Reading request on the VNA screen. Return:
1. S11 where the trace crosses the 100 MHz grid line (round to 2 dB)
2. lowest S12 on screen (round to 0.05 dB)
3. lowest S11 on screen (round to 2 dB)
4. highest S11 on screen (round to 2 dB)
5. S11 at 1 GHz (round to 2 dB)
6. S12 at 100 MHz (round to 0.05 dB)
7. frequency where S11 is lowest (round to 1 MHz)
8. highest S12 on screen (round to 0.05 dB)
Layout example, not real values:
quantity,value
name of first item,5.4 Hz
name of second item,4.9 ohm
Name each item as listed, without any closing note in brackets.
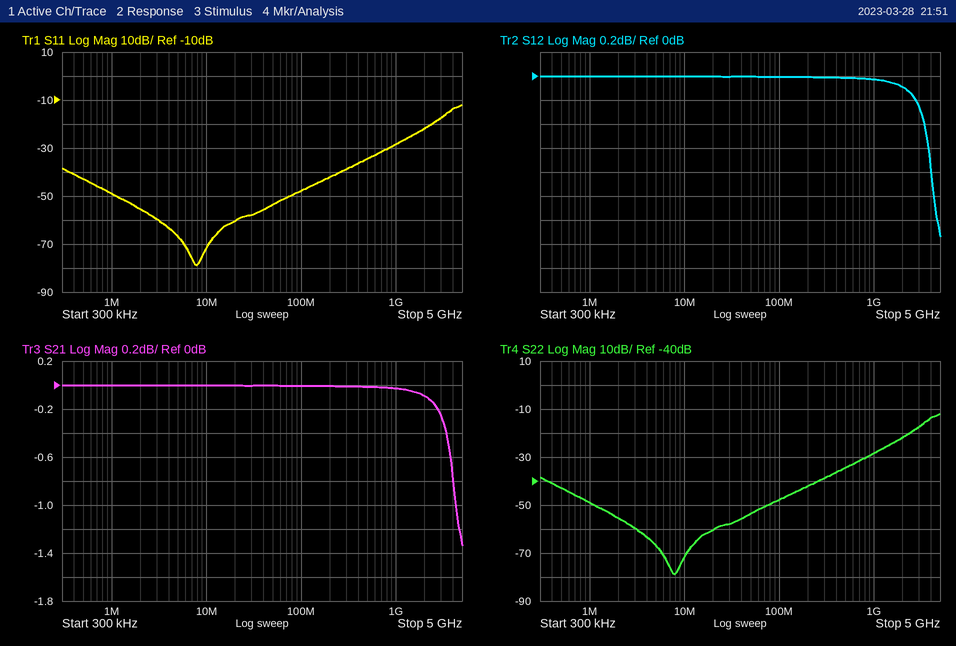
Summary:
quantity,value
S11 where the trace crosses the 100 MHz grid line,-48 dB
lowest S12 on screen,-1.35 dB
lowest S11 on screen,-78 dB
highest S11 on screen,-12 dB
S11 at 1 GHz,-28 dB
S12 at 100 MHz,0.00 dB
frequency where S11 is lowest,8 MHz
highest S12 on screen,0.00 dB
